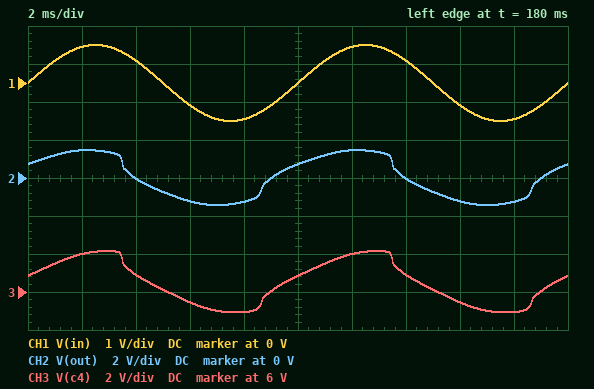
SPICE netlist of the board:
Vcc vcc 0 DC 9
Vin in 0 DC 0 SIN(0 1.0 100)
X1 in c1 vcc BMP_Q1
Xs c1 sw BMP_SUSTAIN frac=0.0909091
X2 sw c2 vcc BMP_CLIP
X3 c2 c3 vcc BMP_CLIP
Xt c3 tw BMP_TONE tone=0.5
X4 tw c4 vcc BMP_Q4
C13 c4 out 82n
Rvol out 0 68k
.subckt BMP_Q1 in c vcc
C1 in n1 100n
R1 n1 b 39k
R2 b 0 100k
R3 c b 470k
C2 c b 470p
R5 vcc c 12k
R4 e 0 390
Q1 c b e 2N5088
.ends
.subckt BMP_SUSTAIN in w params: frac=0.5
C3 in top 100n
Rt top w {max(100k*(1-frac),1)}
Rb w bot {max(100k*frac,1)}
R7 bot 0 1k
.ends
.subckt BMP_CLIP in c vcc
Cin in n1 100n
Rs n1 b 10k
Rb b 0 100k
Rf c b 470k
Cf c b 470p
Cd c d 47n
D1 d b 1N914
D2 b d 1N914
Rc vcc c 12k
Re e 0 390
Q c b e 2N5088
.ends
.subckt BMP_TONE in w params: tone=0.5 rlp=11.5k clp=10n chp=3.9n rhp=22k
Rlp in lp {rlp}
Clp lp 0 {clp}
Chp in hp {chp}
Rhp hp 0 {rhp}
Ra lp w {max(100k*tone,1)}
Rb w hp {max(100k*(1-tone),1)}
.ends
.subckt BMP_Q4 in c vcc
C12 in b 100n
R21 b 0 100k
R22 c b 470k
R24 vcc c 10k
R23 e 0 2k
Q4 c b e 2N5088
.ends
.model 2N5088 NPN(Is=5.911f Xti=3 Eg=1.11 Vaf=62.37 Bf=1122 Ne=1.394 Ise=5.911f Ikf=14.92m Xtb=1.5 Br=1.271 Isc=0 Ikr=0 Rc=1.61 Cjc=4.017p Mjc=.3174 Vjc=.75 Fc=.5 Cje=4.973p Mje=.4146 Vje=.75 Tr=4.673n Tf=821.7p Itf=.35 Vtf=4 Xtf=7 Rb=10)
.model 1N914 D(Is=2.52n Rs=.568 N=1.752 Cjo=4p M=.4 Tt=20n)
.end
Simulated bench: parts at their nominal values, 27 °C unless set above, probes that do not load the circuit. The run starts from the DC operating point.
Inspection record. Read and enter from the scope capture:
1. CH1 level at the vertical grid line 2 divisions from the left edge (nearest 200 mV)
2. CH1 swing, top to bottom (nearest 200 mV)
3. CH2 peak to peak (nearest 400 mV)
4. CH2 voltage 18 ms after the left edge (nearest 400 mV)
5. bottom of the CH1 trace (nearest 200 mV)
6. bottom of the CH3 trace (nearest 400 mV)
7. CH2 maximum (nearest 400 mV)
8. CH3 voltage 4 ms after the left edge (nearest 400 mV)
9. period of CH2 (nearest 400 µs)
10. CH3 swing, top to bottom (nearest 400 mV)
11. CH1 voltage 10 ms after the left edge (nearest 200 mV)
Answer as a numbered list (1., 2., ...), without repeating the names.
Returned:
1. 600 mV
2. 2.0 V
3. 2.8 V
4. -1.2 V
5. -1.0 V
6. 4.8 V
7. 1.6 V
8. 6.8 V
9. 10.0 ms
10. 3.2 V
11. 0 V
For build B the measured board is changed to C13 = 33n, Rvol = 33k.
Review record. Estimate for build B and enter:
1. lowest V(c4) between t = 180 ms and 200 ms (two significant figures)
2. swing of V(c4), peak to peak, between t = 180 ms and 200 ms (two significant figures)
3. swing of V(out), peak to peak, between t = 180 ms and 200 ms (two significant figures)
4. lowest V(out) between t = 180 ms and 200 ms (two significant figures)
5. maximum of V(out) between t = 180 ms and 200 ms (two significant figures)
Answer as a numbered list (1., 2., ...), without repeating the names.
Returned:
1. 4.9 V
2. 3.4 V
3. 1.6 V
4. -810 mV
5. 800 mV
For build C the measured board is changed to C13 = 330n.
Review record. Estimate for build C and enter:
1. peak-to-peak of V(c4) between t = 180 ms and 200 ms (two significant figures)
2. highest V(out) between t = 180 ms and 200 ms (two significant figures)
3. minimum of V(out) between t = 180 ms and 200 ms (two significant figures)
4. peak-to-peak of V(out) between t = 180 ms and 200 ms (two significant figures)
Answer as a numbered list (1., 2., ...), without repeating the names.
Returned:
1. 3.2 V
2. 1.6 V
3. -1.5 V
4. 3.1 V
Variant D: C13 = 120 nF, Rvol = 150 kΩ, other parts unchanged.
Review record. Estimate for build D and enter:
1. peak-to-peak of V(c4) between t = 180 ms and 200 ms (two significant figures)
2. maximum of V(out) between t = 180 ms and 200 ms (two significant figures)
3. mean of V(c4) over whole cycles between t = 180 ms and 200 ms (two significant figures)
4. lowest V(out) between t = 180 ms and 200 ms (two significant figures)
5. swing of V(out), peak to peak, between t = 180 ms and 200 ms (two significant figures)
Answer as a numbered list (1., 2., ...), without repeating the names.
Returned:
1. 3.4 V
2. 1.7 V
3. 6.5 V
4. -1.6 V
5. 3.3 V
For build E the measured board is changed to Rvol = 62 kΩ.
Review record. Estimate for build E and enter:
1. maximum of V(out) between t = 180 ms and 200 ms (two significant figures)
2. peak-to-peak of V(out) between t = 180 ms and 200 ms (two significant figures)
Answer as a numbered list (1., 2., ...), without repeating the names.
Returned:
1. 1.4 V
2. 2.8 V
